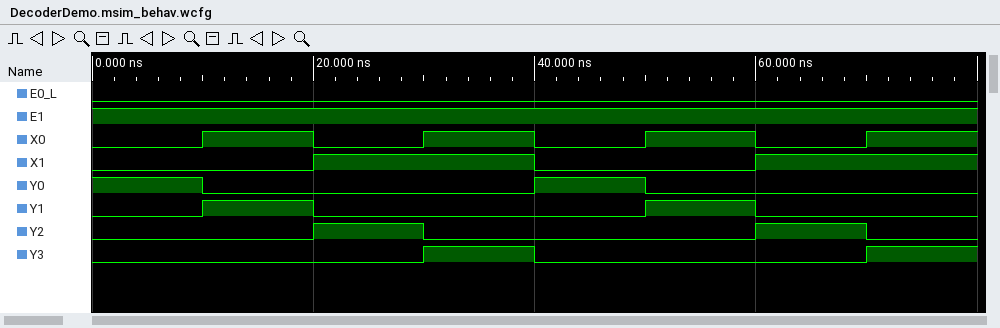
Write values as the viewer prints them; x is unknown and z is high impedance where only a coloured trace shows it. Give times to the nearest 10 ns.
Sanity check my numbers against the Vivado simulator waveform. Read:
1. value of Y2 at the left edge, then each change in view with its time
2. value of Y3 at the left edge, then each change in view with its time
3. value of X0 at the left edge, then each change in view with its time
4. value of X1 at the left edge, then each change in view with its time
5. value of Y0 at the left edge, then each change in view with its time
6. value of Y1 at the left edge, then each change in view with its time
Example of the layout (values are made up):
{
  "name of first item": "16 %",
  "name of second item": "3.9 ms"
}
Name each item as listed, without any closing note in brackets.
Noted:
{
  "value of Y2 at the left edge, then each change in view with its time": "0, 1 at 20 ns, 0 at 30 ns, 1 at 60 ns, 0 at 70 ns",
  "value of Y3 at the left edge, then each change in view with its time": "0, 1 at 30 ns, 0 at 40 ns, 1 at 70 ns",
  "value of X0 at the left edge, then each change in view with its time": "0, 1 at 10 ns, 0 at 20 ns, 1 at 30 ns, 0 at 40 ns, 1 at 50 ns, 0 at 60 ns, 1 at 70 ns",
  "value of X1 at the left edge, then each change in view with its time": "0, 1 at 20 ns, 0 at 40 ns, 1 at 60 ns",
  "value of Y0 at the left edge, then each change in view with its time": "1, 0 at 10 ns, 1 at 40 ns, 0 at 50 ns",
  "value of Y1 at the left edge, then each change in view with its time": "0, 1 at 10 ns, 0 at 20 ns, 1 at 50 ns, 0 at 60 ns"
}
